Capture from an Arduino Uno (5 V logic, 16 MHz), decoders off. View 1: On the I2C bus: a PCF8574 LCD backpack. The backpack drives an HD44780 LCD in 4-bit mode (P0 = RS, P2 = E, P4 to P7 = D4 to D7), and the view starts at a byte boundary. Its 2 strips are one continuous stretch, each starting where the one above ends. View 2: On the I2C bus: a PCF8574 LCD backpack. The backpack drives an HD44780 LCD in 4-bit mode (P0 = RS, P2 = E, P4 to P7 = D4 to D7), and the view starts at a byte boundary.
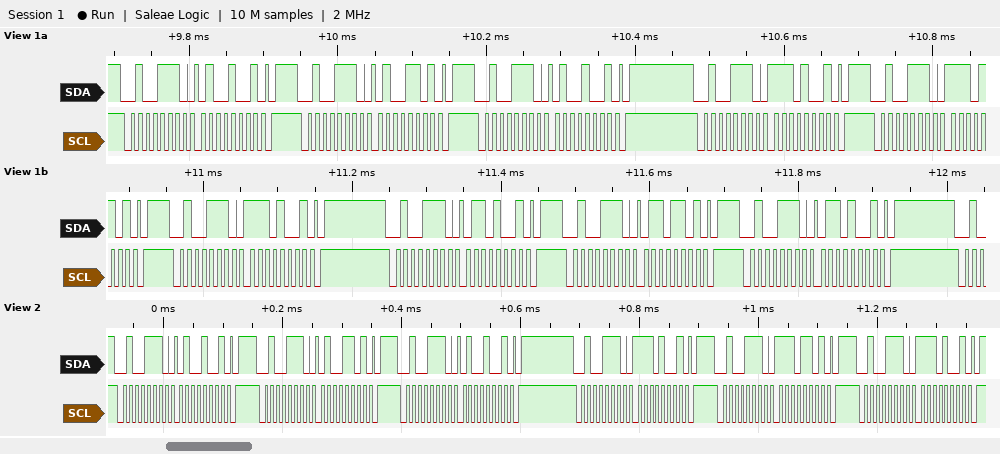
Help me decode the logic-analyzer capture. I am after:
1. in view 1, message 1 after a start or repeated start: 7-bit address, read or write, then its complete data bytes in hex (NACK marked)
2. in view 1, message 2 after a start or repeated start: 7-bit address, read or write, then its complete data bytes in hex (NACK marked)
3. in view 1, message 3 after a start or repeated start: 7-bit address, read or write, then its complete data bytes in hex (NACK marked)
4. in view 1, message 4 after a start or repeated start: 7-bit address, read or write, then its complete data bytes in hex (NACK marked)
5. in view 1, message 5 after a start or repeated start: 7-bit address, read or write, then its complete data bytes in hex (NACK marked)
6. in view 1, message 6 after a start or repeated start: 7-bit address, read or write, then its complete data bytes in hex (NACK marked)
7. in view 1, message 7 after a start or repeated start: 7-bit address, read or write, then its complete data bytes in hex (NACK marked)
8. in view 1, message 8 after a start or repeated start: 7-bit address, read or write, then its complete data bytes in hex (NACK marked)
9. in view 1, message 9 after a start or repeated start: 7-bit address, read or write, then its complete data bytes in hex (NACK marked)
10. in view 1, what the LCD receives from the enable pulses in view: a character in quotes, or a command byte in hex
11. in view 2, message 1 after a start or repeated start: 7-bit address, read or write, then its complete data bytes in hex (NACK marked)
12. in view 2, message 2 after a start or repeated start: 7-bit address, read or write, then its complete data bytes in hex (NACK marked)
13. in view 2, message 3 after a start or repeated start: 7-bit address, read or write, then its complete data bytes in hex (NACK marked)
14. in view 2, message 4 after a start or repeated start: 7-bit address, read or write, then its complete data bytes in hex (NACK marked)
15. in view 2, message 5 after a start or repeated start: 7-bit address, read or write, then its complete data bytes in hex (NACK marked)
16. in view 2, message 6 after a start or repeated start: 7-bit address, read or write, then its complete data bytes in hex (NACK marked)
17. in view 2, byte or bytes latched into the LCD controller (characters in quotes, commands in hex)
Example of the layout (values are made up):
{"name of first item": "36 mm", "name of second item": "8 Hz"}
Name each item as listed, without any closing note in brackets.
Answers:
{"in view 1, message 1 after a start or repeated start: 7-bit address, read or write, then its complete data bytes in hex": "0x27 write: 49", "in view 1, message 2 after a start or repeated start: 7-bit address, read or write, then its complete data bytes in hex": "0x27 write: 4D", "in view 1, message 3 after a start or repeated start: 7-bit address, read or write, then its complete data bytes in hex": "0x27 write: 49", "in view 1, message 4 after a start or repeated start: 7-bit address, read or write, then its complete data bytes in hex": "0x27 write: E9", "in view 1, message 5 after a start or repeated start: 7-bit address, read or write, then its complete data bytes in hex": "0x27 write: ED", "in view 1, message 6 after a start or repeated start: 7-bit address, read or write, then its complete data bytes in hex": "0x27 write: E9", "in view 1, message 7 after a start or repeated start: 7-bit address, read or write, then its complete data bytes in hex": "0x27 write: 69", "in view 1, message 8 after a start or repeated start: 7-bit address, read or write, then its complete data bytes in hex": "0x27 write: 6D", "in view 1, message 9 after a start or repeated start: 7-bit address, read or write, then its complete data bytes in hex": "0x27 write: 69", "in view 1, what the LCD receives from the enable pulses in view: a character in quotes, or a command byte in hex": "'N'", "in view 2, message 1 after a start or repeated start: 7-bit address, read or write, then its complete data bytes in hex": "0x27 write: 49", "in view 2, message 2 after a start or repeated start: 7-bit address, read or write, then its complete data bytes in hex": "0x27 write: 4D", "in view 2, message 3 after a start or repeated start: 7-bit address, read or write, then its complete data bytes in hex": "0x27 write: 49", "in view 2, message 4 after a start or repeated start: 7-bit address, read or write, then its complete data bytes in hex": "0x27 write: E9", "in view 2, message 5 after a start or repeated start: 7-bit address, read or write, then its complete data bytes in hex": "0x27 write: ED", "in view 2, message 6 after a start or repeated start: 7-bit address, read or write, then its complete data bytes in hex": "0x27 write: E9", "in view 2, byte or bytes latched into the LCD controller": "'N'"}
